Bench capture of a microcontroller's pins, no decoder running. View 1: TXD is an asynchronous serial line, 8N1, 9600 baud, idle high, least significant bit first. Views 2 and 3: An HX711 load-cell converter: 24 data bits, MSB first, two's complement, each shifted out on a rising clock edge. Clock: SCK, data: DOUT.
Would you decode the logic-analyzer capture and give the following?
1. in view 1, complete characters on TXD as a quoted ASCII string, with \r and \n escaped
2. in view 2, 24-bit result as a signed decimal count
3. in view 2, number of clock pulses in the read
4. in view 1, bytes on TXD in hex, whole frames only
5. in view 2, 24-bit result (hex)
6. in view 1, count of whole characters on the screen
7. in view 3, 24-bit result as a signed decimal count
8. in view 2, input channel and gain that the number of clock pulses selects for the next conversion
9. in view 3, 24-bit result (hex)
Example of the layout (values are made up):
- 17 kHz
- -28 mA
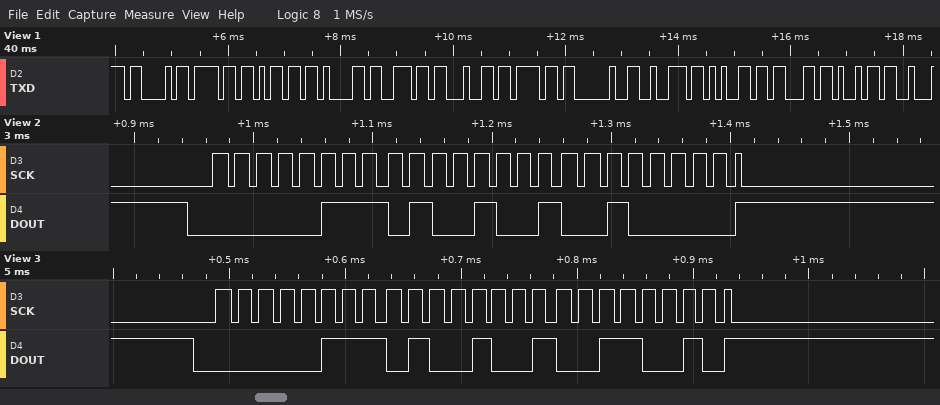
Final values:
- "Comando reci"
- 477472
- 25
- 0x43 0x6F 0x6D 0x61 0x6E 0x64 0x6F 0x20 0x72 0x65 0x63 0x69
- 0x074920
- 12
- 477490
- channel A, gain 128
- 0x074932
